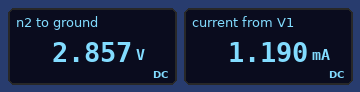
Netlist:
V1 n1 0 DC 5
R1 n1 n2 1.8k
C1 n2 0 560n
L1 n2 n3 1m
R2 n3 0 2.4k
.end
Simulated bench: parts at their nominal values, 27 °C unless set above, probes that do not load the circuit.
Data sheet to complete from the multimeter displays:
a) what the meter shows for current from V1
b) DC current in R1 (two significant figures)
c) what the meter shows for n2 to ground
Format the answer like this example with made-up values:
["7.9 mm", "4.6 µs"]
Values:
["1.190 mA", "1.2 mA", "2.857 V"]
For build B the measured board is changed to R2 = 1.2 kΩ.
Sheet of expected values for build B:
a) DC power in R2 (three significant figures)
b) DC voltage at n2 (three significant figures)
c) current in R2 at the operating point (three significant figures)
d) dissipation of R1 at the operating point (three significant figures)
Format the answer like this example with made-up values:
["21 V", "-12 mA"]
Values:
["3.33 mW", "2.00 V", "1.67 mA", "5.00 mW"]
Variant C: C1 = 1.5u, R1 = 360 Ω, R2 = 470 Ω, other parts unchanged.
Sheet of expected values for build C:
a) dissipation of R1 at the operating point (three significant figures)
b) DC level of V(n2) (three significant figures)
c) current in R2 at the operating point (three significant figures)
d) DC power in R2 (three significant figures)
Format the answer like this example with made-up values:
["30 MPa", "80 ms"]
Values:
["13.1 mW", "2.83 V", "6.02 mA", "17.1 mW"]
